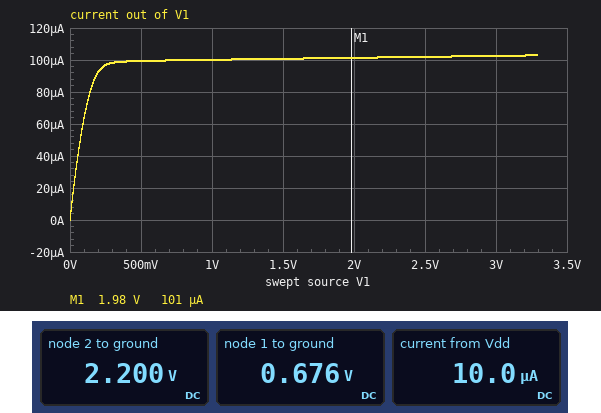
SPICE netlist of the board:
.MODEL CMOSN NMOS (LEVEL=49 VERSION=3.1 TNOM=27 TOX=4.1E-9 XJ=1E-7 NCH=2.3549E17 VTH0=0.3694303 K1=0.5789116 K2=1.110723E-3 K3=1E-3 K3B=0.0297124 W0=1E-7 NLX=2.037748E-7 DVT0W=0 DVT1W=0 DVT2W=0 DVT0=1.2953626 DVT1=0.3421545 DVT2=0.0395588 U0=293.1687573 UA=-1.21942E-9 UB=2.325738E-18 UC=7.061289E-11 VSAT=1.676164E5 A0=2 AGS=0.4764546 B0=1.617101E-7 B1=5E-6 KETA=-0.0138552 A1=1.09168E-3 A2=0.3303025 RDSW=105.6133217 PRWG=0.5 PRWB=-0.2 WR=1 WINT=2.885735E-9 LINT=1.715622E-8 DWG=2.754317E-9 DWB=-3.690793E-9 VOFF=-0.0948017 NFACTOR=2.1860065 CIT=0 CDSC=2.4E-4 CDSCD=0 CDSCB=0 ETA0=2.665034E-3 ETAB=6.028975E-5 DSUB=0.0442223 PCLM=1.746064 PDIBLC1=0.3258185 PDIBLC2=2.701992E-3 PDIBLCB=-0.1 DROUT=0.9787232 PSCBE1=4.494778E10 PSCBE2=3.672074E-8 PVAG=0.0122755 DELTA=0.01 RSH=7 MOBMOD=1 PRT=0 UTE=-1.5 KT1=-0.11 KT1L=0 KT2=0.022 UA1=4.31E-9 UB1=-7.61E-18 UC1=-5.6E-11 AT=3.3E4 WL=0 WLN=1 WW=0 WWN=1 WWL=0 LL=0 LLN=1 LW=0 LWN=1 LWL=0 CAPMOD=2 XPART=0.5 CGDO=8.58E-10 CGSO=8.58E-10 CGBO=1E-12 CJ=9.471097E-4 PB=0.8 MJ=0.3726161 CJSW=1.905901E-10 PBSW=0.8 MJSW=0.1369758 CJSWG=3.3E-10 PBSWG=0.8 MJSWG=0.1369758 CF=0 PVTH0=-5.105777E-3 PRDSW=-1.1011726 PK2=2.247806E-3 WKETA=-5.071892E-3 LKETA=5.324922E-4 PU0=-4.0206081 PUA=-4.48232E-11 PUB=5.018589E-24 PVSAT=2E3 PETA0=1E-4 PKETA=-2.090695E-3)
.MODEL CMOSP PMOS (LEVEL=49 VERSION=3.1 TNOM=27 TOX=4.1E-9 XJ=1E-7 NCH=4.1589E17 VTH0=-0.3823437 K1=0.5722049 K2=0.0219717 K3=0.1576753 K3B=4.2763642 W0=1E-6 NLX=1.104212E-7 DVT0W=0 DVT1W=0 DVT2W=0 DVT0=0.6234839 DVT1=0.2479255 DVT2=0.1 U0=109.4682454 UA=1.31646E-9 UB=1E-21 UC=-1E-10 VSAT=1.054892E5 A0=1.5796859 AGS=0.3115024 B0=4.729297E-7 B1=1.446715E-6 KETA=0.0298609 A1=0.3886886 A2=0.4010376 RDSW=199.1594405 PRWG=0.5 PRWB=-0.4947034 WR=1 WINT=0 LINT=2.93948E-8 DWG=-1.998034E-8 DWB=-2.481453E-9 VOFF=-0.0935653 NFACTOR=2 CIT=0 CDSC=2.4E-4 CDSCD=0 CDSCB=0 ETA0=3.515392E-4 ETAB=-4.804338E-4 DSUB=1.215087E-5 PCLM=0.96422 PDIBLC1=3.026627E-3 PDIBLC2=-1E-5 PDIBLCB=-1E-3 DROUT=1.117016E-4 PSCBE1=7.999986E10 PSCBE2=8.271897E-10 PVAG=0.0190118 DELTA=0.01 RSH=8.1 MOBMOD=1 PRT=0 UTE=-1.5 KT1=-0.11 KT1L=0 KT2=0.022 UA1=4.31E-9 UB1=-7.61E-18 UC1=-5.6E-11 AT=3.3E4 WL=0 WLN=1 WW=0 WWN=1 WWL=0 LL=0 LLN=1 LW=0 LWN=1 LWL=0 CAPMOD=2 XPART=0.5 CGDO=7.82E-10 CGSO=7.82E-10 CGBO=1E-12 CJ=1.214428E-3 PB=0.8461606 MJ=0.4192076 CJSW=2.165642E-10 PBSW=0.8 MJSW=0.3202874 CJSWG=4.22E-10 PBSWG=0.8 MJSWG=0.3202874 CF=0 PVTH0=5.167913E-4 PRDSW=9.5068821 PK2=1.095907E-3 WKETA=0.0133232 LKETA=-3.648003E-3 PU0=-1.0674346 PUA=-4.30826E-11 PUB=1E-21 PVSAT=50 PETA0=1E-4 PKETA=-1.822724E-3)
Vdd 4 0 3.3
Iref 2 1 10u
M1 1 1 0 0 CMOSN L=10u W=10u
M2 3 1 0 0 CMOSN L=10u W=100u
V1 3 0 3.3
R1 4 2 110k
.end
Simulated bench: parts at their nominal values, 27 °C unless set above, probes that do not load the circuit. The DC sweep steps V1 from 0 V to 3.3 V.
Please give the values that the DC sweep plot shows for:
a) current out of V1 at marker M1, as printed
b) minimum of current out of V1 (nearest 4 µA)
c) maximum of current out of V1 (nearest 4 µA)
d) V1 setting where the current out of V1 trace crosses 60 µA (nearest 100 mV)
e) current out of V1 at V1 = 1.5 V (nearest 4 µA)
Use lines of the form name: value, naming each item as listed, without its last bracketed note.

current out of V1 at marker M1, as printed: 101 µA
minimum of current out of V1: 0 A
maximum of current out of V1: 104 µA
V1 setting where the current out of V1 trace crosses 60 µA: 100 mV
current out of V1 at V1 = 1.5 V: 100 µA
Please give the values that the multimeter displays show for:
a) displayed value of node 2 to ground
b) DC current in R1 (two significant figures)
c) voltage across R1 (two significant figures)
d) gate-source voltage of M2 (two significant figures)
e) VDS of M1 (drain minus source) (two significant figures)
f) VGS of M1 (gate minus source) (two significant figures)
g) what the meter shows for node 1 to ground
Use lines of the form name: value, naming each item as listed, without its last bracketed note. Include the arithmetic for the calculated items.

displayed value of node 2 to ground: 2.200 V
DC current in R1: (3.3 V - 2.2 V) / 110 kΩ = 10 µA
voltage across R1: 3.3 V - 2.2 V = 1.1 V
gate-source voltage of M2: 676 mV = 680 mV
VDS of M1 (drain minus source): 676 mV = 680 mV
VGS of M1 (gate minus source): 676 mV = 680 mV
what the meter shows for node 1 to ground: 0.676 V
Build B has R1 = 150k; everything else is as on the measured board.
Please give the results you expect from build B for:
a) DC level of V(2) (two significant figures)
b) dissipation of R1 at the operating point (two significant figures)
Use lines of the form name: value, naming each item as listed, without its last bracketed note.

DC level of V(2): 1.8 V
dissipation of R1 at the operating point: 15 µW
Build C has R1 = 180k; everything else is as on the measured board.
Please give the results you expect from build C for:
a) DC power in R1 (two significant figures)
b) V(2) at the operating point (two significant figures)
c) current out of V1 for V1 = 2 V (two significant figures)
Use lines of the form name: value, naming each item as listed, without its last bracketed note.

DC power in R1: 18 µW
V(2) at the operating point: 1.5 V
current out of V1 for V1 = 2 V: 100 µA
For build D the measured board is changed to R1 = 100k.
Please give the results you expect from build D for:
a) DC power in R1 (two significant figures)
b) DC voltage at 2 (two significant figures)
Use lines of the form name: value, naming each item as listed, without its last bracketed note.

DC power in R1: 10 µW
DC voltage at 2: 2.3 V
